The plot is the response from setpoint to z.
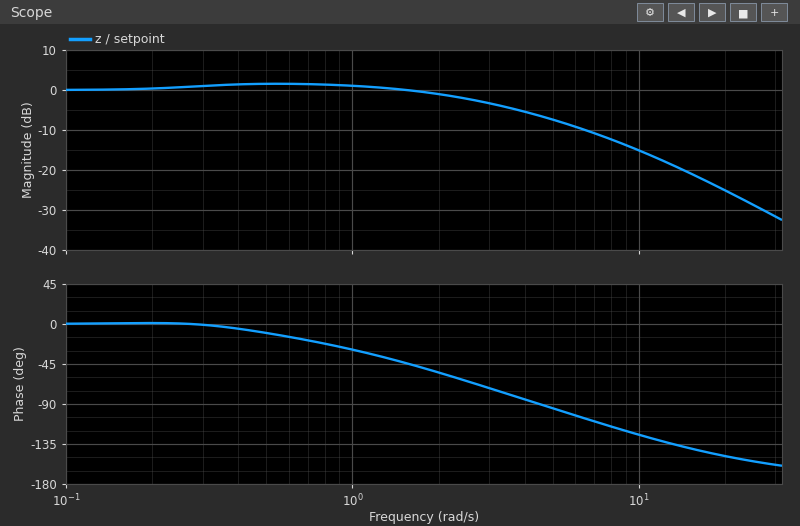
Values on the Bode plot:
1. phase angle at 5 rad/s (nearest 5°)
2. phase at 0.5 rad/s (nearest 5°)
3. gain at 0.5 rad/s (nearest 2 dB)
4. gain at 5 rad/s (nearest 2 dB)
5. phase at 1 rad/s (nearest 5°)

-95°
-10°
2 dB
-8 dB
-30°
